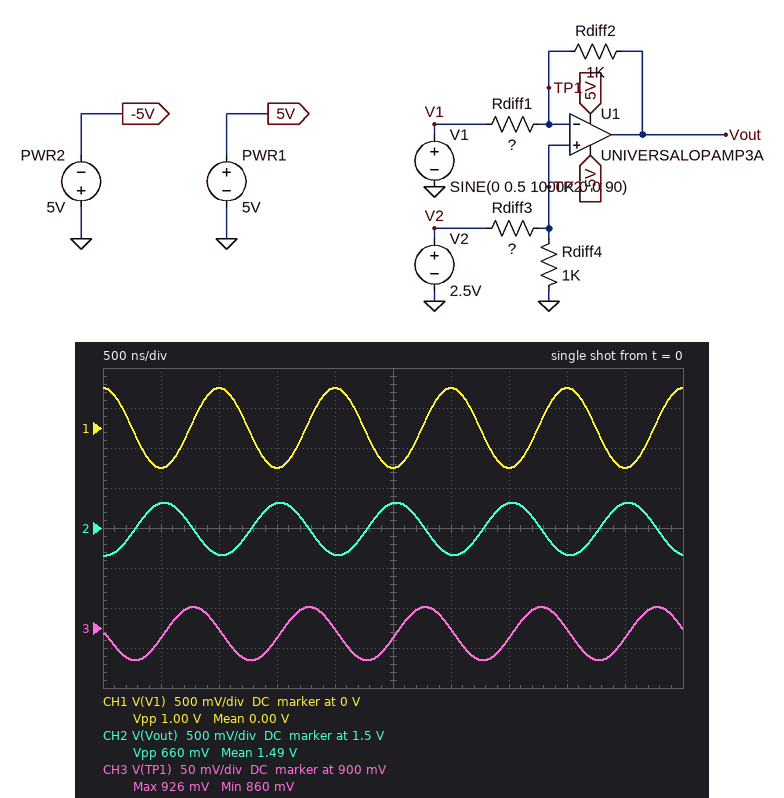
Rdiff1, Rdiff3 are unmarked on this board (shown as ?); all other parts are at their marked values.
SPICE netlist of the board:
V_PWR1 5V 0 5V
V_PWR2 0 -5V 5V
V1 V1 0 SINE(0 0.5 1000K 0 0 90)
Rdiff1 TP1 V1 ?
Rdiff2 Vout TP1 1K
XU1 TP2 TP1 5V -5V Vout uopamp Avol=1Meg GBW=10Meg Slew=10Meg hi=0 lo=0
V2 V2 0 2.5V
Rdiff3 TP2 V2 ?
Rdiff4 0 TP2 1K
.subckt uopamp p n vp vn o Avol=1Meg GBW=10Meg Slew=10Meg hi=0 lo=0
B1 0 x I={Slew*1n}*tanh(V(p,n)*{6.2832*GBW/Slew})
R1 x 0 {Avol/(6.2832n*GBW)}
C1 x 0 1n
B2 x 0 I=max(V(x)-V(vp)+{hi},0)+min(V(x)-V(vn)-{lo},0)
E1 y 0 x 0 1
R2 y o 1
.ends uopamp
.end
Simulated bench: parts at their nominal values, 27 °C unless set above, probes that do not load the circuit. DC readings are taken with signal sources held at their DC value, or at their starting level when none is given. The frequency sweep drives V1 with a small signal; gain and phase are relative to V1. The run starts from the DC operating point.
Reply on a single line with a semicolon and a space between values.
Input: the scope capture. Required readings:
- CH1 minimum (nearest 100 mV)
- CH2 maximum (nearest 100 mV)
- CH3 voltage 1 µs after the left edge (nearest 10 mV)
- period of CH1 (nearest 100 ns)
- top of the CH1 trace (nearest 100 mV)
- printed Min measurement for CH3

-500 mV; 1.8 V; 900 mV; 1.0 µs; 500 mV; 860 mV
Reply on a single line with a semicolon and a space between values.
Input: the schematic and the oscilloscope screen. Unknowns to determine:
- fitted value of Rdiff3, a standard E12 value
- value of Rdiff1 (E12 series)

1.8 kΩ; 1.5 kΩ
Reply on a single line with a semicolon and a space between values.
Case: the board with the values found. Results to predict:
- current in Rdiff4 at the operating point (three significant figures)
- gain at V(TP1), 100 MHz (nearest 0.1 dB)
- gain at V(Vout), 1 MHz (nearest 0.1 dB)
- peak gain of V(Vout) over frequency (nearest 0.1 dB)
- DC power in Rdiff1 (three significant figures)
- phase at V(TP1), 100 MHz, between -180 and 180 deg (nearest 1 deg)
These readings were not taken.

893 µA; -8.0 dB; -3.6 dB; -3.5 dB; 103 µW; 3 deg
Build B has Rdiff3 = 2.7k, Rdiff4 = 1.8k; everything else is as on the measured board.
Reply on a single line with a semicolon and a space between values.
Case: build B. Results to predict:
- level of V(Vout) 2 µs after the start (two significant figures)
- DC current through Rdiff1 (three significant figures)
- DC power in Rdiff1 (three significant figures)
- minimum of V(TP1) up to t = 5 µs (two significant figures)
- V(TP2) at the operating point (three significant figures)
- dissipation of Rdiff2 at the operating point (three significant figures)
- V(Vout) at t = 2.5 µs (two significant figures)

1.3 V; 333 µA; 167 µW; 970 mV; 1.00 V; 111 µW; 2.0 V
